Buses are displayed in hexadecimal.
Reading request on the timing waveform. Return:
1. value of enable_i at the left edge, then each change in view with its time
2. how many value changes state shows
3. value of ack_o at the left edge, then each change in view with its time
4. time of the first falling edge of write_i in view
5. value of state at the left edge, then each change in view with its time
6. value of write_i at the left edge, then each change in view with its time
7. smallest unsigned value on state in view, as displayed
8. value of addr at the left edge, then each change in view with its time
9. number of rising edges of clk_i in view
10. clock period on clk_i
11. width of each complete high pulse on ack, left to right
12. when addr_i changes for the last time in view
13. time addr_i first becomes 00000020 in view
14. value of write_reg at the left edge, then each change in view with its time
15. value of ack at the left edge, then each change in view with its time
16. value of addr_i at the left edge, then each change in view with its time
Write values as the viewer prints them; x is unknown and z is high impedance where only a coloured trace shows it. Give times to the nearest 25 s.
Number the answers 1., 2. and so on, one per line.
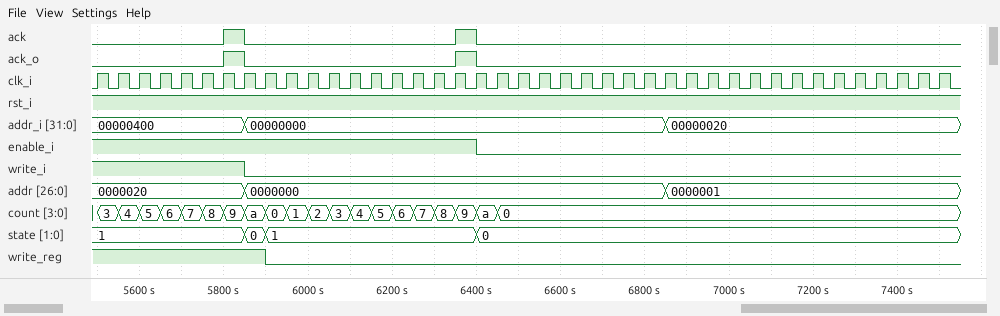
1. 1, 0 at 6400 s
2. 3
3. 0, 1 at 5800 s, 0 at 5850 s, 1 at 6350 s, 0 at 6400 s
4. 5850 s
5. 1, 0 at 5850 s, 1 at 5900 s, 0 at 6400 s
6. 1, 0 at 5850 s
7. 0
8. 0000020, 0000000 at 5850 s, 0000001 at 6850 s
9. 41
10. 50 s
11. 50 s, 50 s
12. 6850 s
13. 6850 s
14. 1, 0 at 5900 s
15. 0, 1 at 5800 s, 0 at 5850 s, 1 at 6350 s, 0 at 6400 s
16. 00000400, 00000000 at 5850 s, 00000020 at 6850 s
